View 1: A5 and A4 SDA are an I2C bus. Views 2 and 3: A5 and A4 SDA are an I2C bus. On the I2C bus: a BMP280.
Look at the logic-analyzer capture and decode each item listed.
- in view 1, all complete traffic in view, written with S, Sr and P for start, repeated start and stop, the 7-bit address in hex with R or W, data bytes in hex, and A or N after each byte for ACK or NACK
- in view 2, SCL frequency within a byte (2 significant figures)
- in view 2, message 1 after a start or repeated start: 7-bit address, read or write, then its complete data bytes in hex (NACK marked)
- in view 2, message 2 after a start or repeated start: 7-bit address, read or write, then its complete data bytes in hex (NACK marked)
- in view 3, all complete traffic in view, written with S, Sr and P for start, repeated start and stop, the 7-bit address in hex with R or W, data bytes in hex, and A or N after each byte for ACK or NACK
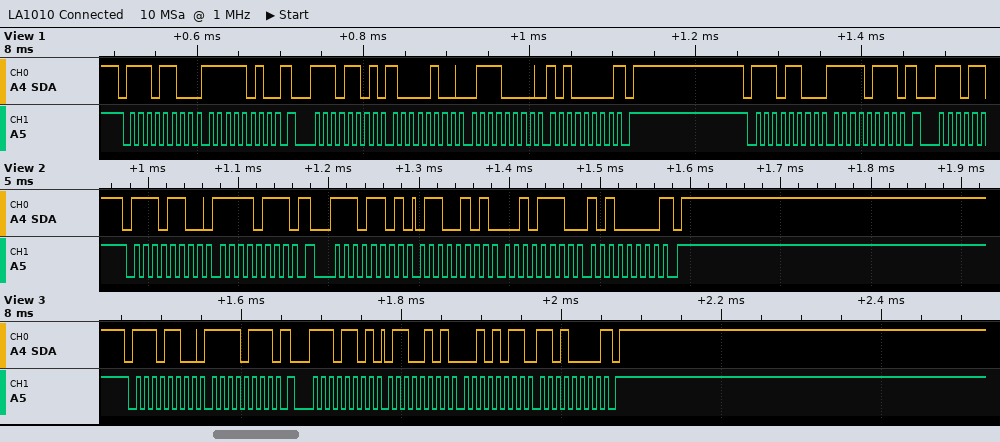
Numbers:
S 76W A FA A Sr 76R A 84 A 70 A A0 N P S 76W A F7 A
100 kHz
0x76 write: F7
0x76 read: 65 2E A0 NACK
S 76W A F7 A Sr 76R A 65 A 2B A D0 N P
